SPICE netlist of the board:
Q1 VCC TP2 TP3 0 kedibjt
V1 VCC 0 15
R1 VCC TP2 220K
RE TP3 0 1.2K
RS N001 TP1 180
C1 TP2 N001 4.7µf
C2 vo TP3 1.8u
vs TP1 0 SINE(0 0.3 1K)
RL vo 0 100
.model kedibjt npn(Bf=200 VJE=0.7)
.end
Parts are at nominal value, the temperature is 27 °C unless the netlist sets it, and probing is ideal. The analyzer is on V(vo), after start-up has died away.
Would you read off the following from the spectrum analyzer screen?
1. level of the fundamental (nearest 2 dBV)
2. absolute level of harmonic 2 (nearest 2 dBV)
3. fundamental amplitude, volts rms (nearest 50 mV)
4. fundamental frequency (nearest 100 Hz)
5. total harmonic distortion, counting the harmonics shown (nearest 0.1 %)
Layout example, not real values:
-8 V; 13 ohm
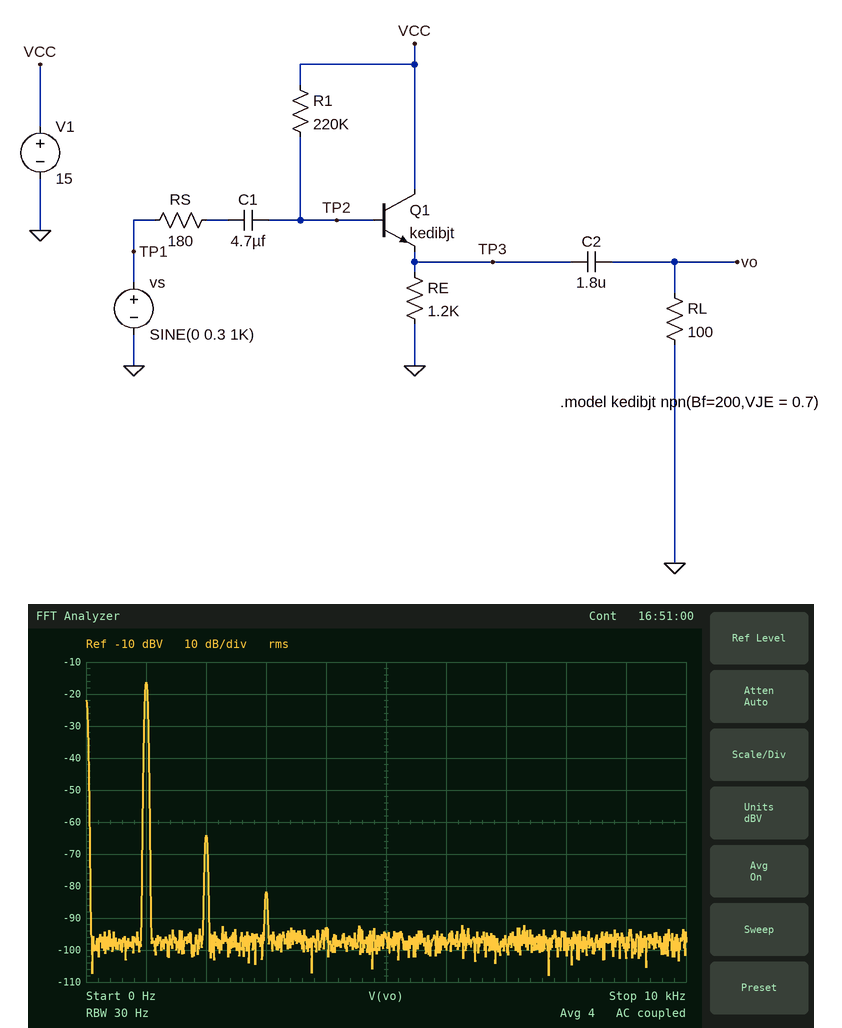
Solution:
-16 dBV; -64 dBV; 150 mV; 1.0 kHz; 0.4 %
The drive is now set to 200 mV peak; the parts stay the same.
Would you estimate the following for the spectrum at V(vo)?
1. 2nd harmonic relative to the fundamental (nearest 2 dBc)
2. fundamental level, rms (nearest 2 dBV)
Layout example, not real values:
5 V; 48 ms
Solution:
-52 dBc; -20 dBV
